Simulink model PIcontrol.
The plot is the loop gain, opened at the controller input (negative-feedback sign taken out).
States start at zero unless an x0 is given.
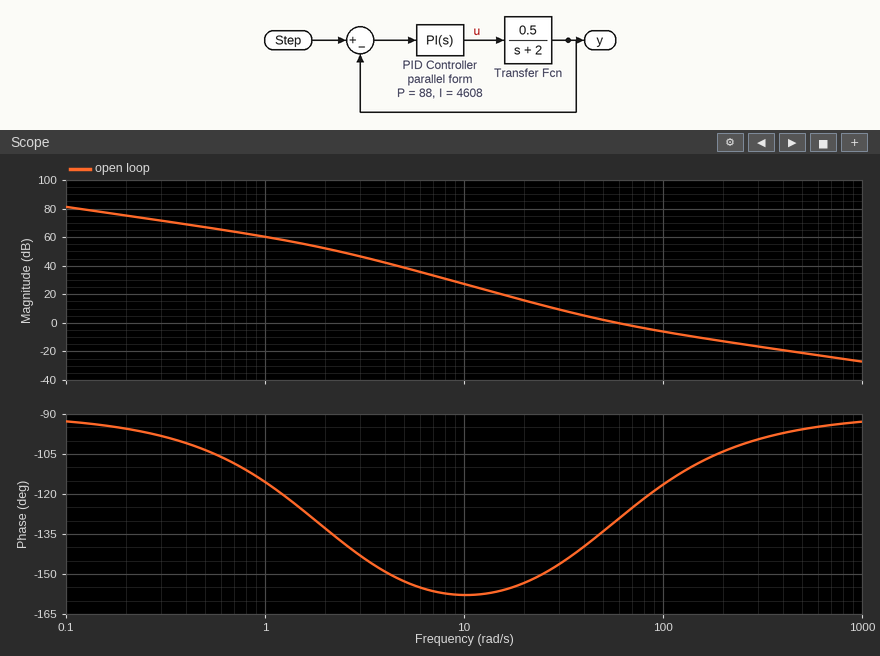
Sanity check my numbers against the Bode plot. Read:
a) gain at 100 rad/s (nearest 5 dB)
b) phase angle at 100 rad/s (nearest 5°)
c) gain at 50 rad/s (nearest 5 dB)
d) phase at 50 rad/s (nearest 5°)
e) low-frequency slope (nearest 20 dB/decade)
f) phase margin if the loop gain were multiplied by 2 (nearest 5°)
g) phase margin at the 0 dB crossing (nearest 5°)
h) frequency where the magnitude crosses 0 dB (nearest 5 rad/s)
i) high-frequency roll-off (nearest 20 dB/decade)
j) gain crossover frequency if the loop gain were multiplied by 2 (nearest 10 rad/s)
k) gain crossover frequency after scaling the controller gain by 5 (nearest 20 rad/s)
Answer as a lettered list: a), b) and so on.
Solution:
a) -5 dB
b) -115°
c) 0 dB
d) -135°
e) -20 dB/decade
f) 65°
g) 50°
h) 60 rad/s
i) -20 dB/decade
j) 100 rad/s
k) 220 rad/s
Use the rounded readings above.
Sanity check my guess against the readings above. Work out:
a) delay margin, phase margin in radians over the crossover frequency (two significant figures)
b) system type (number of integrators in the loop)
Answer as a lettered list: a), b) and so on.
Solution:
a) 0.015 s
b) 1
